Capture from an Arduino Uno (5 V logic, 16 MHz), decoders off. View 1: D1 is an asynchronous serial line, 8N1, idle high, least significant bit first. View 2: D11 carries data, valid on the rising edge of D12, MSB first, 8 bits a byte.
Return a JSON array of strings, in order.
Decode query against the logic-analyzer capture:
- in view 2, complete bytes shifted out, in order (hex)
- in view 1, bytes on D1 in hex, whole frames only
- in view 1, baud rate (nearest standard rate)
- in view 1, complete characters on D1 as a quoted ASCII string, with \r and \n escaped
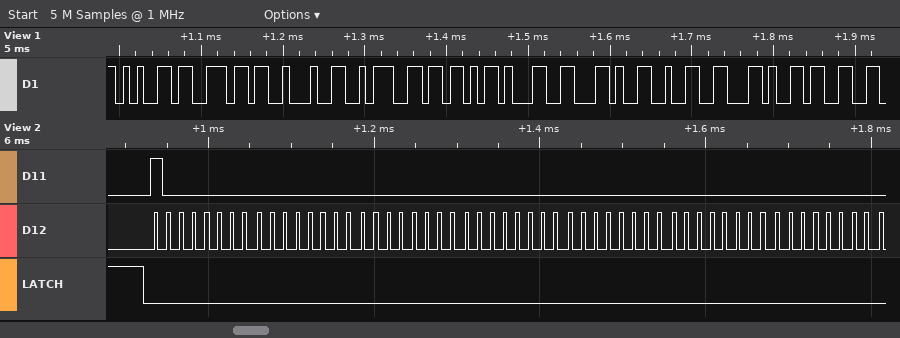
["80 00 00 00 00 00 00", "65 6E 22 3A 5B 31 2C 32 2C 33", "115200 baud", "\"en\\\":[1,2,3\""]
